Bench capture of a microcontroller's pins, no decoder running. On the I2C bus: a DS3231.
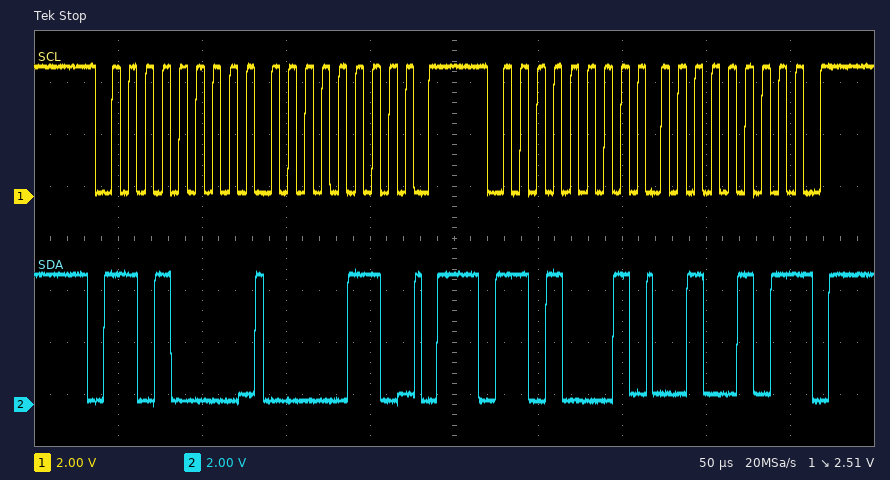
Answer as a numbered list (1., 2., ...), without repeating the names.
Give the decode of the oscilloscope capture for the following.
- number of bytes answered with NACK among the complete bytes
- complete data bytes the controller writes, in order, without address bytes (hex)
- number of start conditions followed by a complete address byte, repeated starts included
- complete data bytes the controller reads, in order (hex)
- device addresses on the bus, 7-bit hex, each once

1. 1
2. 06
3. 2
4. 25
5. 0x68
